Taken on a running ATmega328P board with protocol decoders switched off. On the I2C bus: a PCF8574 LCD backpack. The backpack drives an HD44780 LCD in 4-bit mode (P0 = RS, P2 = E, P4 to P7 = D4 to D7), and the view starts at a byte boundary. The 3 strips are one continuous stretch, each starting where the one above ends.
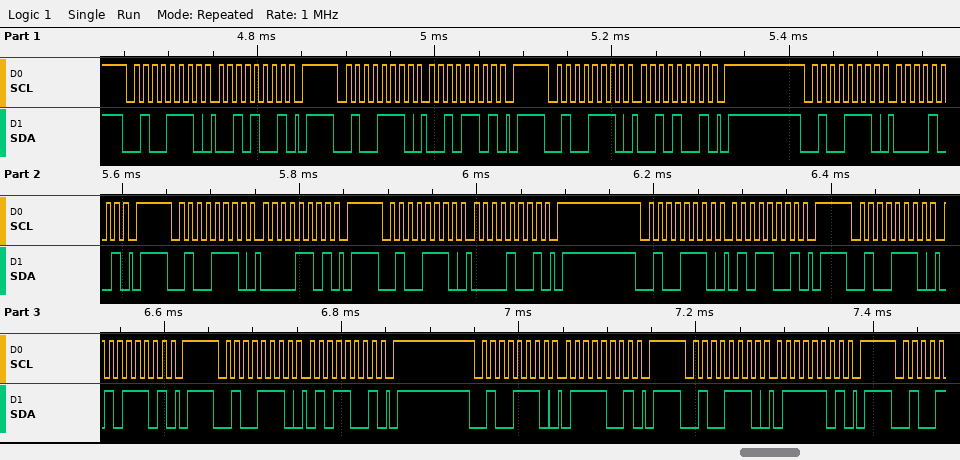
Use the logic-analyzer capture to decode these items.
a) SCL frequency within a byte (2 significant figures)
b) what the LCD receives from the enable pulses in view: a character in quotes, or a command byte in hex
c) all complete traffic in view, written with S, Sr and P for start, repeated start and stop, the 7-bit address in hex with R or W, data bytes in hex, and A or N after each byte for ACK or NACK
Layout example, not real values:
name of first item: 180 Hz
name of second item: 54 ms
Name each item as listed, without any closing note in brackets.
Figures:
SCL frequency within a byte: 100 kHz
what the LCD receives from the enable pulses in view: a character in quotes, or a command byte in hex: ' '
all complete traffic in view, written with S, Sr and P for start, repeated start and stop, the 7-bit address in hex with R or W, data bytes in hex, and A or N after each byte for ACK or NACK: S 27W A 29 A P S 27W A 2D A P S 27W A 29 A P S 27W A 09 A P S 27W A 0D A P S 27W A 09 A P S 27W A 59 A P S 27W A 5D A P S 27W A 59 A P S 27W A 79 A P S 27W A 7D A P
